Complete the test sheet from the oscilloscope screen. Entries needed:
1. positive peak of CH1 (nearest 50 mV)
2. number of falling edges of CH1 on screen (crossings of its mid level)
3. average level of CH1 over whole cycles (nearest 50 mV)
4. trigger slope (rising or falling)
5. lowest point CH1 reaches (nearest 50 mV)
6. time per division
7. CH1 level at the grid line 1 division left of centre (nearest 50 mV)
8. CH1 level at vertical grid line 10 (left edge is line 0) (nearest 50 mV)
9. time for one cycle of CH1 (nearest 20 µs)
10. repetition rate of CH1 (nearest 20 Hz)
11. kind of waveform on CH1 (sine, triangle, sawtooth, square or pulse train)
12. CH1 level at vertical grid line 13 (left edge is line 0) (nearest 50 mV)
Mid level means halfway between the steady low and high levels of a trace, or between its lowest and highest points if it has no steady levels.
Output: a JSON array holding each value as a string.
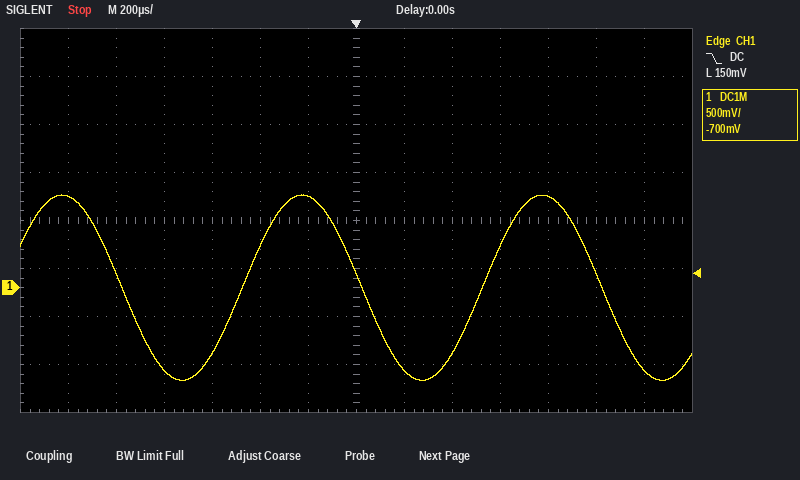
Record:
["950 mV", "3", "0 mV", "falling", "-950 mV", "200 µs", "950 mV", "450 mV", "1.00 ms", "1.00 kHz", "sine", "-850 mV"]
